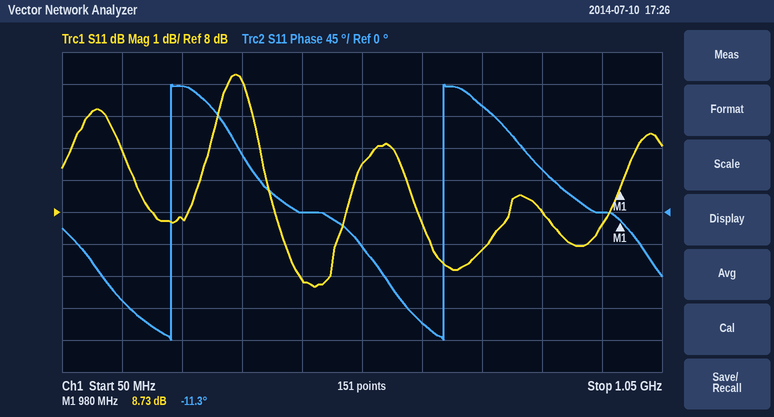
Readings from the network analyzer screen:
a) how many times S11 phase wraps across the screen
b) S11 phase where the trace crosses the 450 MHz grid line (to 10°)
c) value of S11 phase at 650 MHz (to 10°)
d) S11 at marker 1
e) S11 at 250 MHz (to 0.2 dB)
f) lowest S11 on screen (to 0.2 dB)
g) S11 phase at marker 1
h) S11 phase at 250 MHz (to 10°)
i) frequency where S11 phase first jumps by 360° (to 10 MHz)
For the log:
2
0°
-160°
8.73 dB
7.8 dB
5.6 dB
-11.3°
180°
230 MHz
